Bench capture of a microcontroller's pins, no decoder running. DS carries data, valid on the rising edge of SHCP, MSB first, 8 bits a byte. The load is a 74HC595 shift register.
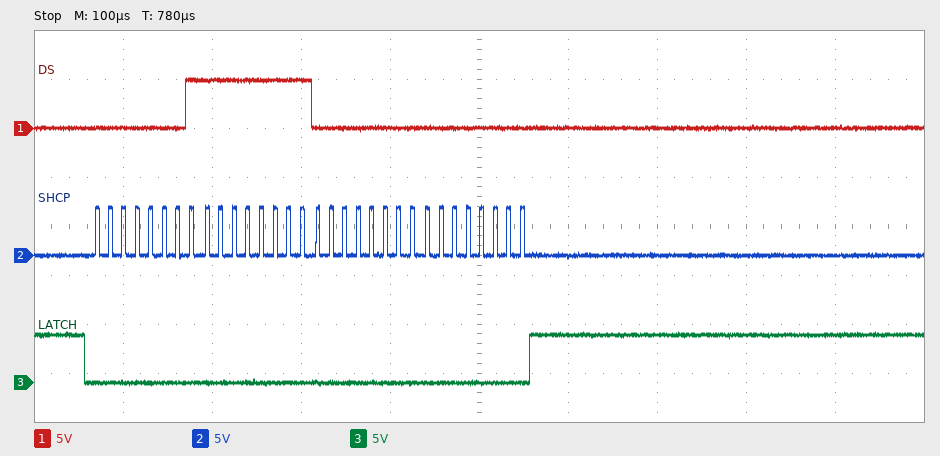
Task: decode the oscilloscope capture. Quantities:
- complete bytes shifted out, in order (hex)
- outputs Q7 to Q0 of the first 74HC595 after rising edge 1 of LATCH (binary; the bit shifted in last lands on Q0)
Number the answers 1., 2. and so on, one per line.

1. 01 FF 00 00
2. 00000000
